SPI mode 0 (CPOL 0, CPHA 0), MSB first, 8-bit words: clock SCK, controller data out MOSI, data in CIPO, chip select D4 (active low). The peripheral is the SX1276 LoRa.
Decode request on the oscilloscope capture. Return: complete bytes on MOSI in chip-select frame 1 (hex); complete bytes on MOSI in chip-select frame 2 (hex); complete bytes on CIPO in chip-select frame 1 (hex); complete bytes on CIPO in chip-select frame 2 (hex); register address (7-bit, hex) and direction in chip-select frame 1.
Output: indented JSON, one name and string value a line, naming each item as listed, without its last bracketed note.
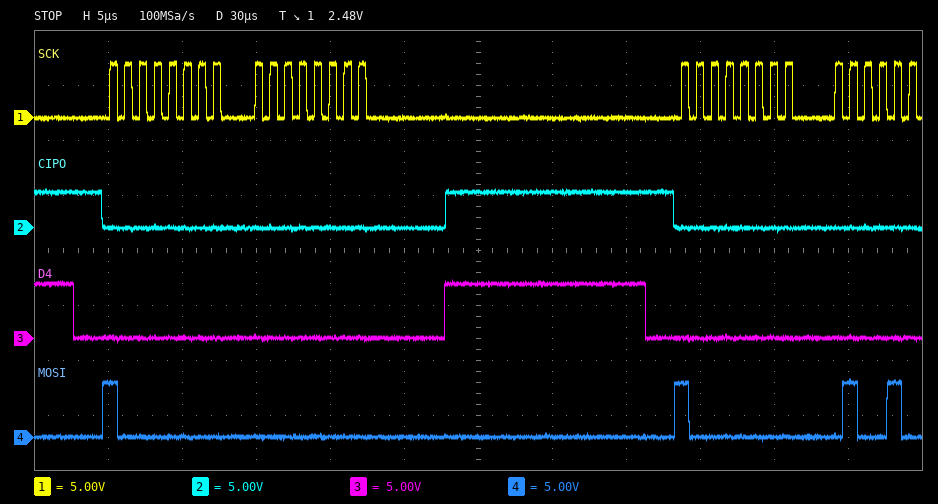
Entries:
{
  "complete bytes on MOSI in chip-select frame 1": "80 00",
  "complete bytes on MOSI in chip-select frame 2": "80",
  "complete bytes on CIPO in chip-select frame 1": "00 00",
  "complete bytes on CIPO in chip-select frame 2": "00",
  "register address (7-bit, hex) and direction in chip-select frame 1": "0x00 write"
}
